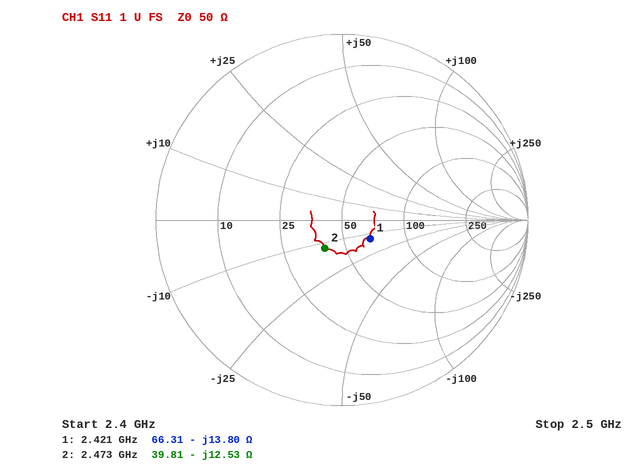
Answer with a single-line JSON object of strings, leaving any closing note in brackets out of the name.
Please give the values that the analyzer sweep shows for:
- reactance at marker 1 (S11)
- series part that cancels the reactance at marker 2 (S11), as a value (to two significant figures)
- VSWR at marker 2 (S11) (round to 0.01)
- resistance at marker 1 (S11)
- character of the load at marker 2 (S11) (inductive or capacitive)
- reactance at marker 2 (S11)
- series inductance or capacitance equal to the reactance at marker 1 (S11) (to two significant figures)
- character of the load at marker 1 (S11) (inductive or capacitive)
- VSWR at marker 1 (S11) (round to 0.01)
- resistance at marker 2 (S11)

{"reactance at marker 1": "-13.80 Ω", "series part that cancels the reactance at marker 2 (S11), as a value": "810 pH", "VSWR at marker 2 (S11)": "1.43", "resistance at marker 1": "66.31 Ω", "character of the load at marker 2 (S11)": "capacitive", "reactance at marker 2": "-12.53 Ω", "series inductance or capacitance equal to the reactance at marker 1 (S11)": "4.8 pF", "character of the load at marker 1 (S11)": "capacitive", "VSWR at marker 1 (S11)": "1.45", "resistance at marker 2": "39.81 Ω"}
